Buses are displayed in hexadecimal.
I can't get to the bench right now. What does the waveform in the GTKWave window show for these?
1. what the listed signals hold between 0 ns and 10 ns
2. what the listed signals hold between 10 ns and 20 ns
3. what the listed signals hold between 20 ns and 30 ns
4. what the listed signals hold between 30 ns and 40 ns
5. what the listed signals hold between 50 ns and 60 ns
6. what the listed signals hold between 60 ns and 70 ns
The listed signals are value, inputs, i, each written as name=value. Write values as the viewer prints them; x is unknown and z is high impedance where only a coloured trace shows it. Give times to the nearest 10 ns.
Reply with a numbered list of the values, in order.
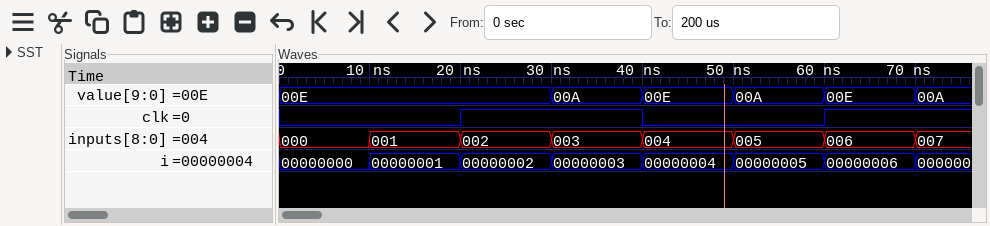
1. value=00E, inputs=000, i=00000000
2. value=00E, inputs=001, i=00000001
3. value=00E, inputs=002, i=00000002
4. value=00A, inputs=003, i=00000003
5. value=00A, inputs=005, i=00000005
6. value=00E, inputs=006, i=00000006
